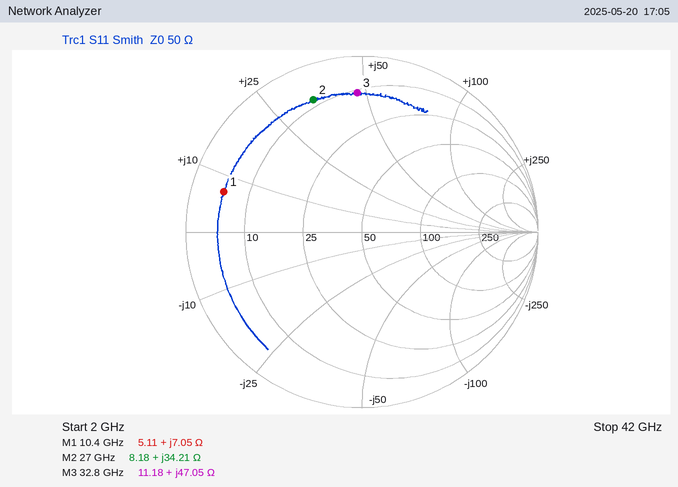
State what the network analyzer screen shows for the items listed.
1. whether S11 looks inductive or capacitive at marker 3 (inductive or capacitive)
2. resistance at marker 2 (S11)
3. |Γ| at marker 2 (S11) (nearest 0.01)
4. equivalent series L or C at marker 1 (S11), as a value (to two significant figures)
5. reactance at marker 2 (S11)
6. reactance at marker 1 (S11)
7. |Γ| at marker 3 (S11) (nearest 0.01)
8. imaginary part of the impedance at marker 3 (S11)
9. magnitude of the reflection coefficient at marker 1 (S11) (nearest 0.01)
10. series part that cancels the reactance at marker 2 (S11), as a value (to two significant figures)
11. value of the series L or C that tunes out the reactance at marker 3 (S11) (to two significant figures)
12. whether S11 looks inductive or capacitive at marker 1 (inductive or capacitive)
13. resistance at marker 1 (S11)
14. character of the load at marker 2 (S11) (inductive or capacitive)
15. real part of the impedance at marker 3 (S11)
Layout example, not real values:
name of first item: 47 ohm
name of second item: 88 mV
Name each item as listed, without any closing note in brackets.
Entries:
whether S11 looks inductive or capacitive at marker 3: inductive
resistance at marker 2: 8.18 Ω
|Γ| at marker 2 (S11): 0.80
equivalent series L or C at marker 1 (S11), as a value: 110 pH
reactance at marker 2: +34.21 Ω
reactance at marker 1: +7.05 Ω
|Γ| at marker 3 (S11): 0.79
imaginary part of the impedance at marker 3: +47.05 Ω
magnitude of the reflection coefficient at marker 1 (S11): 0.82
series part that cancels the reactance at marker 2 (S11), as a value: 170 fF
value of the series L or C that tunes out the reactance at marker 3 (S11): 100 fF
whether S11 looks inductive or capacitive at marker 1: inductive
resistance at marker 1: 5.11 Ω
character of the load at marker 2 (S11): inductive
real part of the impedance at marker 3: 11.18 Ω
